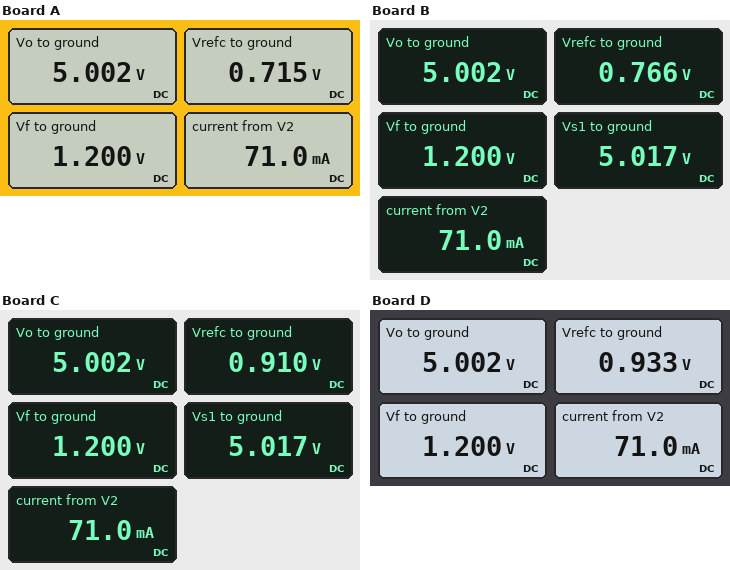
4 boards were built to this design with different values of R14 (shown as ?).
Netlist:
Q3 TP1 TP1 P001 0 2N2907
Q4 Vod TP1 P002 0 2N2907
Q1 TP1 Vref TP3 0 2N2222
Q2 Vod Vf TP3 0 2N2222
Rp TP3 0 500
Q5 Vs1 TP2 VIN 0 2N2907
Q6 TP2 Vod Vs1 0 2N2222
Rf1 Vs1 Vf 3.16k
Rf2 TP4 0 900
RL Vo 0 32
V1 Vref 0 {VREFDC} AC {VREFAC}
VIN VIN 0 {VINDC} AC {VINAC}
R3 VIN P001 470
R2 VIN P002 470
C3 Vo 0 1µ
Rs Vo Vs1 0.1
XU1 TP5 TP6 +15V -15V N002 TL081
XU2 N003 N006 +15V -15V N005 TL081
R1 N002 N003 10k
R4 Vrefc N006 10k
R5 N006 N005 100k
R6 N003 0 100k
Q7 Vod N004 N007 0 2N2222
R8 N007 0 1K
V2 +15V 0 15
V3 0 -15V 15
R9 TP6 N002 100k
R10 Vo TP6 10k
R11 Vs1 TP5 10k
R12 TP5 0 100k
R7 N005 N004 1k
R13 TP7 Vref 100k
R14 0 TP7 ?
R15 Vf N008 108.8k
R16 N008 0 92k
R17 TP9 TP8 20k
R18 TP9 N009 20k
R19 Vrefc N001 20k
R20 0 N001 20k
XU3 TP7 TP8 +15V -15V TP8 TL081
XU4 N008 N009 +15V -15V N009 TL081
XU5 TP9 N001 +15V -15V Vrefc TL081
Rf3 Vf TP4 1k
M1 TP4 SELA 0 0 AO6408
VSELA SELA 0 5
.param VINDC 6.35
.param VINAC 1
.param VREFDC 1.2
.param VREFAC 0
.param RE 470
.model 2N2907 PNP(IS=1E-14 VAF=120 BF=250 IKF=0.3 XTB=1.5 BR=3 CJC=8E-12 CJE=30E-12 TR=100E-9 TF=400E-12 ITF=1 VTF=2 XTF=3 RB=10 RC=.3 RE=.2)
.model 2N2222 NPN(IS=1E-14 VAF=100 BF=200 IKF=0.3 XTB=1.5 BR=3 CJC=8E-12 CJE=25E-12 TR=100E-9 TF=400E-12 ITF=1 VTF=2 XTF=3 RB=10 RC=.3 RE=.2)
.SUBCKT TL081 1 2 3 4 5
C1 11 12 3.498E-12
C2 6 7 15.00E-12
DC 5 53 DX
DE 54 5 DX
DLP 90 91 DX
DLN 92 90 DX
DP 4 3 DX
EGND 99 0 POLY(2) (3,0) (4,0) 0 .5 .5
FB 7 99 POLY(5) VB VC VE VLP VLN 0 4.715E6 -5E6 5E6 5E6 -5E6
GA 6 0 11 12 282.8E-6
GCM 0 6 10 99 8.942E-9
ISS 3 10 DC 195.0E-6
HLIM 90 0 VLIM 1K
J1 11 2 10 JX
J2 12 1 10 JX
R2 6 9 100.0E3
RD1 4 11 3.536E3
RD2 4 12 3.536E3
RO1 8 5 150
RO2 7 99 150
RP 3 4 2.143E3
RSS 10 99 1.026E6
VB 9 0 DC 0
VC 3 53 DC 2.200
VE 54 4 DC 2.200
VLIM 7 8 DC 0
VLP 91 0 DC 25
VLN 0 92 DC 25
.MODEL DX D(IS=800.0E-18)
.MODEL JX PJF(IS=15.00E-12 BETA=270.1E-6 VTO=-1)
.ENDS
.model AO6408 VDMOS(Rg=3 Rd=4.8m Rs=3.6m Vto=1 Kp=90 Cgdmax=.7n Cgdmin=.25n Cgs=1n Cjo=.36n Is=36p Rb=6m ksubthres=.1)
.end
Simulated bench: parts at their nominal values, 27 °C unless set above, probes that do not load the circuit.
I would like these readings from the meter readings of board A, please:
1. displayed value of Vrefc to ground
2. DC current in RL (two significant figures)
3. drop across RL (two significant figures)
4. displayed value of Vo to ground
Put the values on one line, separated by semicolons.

0.715 V; 160 mA; 5.0 V; 5.002 V
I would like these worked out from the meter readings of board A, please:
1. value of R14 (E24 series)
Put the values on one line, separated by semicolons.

16 kΩ
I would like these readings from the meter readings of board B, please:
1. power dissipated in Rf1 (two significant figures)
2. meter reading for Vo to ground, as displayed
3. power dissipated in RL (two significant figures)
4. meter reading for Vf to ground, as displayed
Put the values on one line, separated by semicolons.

4.6 mW; 5.002 V; 780 mW; 1.200 V
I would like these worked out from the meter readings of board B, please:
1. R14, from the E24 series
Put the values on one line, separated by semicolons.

22 kΩ
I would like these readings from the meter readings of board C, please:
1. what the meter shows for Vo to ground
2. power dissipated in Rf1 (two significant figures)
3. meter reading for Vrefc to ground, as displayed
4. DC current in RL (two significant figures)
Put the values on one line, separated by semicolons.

5.002 V; 4.6 mW; 0.910 V; 160 mA
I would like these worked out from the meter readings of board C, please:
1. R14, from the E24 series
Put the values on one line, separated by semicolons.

43 kΩ
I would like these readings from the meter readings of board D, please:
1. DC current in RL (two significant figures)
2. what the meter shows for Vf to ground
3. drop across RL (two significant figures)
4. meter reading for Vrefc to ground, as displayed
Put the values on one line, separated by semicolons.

160 mA; 1.200 V; 5.0 V; 0.933 V
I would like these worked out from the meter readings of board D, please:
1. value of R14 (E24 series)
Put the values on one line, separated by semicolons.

47 kΩ
